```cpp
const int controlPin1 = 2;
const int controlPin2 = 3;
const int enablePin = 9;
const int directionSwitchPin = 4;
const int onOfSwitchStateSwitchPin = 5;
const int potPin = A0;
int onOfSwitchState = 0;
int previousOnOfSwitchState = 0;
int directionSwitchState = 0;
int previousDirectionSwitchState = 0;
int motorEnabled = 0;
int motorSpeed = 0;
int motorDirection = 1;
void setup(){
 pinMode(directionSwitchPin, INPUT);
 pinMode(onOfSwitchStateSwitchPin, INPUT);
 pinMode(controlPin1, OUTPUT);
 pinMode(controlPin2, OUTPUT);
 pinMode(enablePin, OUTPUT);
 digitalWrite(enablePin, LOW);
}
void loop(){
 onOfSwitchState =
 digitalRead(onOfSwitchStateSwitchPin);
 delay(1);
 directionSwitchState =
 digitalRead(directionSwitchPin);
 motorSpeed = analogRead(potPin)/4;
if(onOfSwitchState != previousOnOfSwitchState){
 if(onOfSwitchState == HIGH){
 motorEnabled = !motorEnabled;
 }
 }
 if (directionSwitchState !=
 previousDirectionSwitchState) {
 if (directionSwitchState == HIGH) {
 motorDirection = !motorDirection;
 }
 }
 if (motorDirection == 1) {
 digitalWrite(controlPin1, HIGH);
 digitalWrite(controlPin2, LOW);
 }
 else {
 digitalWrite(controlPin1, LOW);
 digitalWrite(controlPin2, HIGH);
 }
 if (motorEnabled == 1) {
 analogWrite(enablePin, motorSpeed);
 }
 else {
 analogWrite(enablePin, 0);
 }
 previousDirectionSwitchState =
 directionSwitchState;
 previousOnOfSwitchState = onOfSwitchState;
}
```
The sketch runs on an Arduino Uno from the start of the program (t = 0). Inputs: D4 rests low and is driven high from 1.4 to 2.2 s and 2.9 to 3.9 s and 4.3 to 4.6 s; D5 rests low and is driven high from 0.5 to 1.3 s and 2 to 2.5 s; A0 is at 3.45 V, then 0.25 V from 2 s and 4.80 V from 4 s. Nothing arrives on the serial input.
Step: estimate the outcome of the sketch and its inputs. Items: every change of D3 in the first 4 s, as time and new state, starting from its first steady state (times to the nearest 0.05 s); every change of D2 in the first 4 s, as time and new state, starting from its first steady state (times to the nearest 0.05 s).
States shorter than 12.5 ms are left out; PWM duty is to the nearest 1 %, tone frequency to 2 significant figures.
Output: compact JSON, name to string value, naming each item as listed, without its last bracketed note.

{"every change of D3 in the first 4 s, as time and new state, starting from its first steady state": "0 s low; 1.4 s high; 2.9 s low", "every change of D2 in the first 4 s, as time and new state, starting from its first steady state": "0 s high; 1.4 s low; 2.9 s high"}
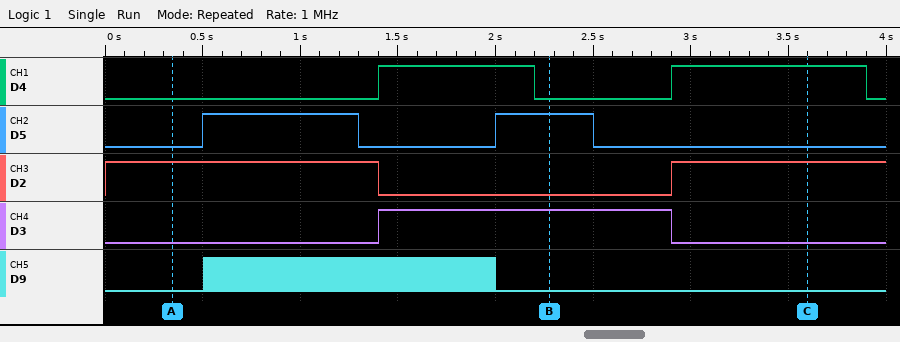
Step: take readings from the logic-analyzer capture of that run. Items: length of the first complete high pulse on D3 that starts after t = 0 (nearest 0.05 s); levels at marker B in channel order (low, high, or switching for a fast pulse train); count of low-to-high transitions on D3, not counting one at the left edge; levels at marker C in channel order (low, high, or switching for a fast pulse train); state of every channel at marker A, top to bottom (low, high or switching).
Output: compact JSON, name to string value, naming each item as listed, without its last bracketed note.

{"length of the first complete high pulse on D3 that starts after t = 0": "1.50 s", "levels at marker B in channel order": "D4 low, D5 high, D2 low, D3 high, D9 low", "count of low-to-high transitions on D3, not counting one at the left edge": "1", "levels at marker C in channel order": "D4 high, D5 low, D2 high, D3 low, D9 low", "state of every channel at marker A, top to bottom": "D4 low, D5 low, D2 high, D3 low, D9 low"}
